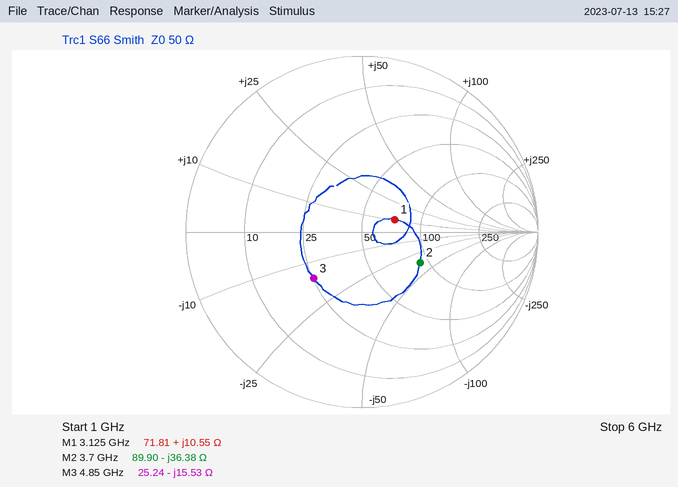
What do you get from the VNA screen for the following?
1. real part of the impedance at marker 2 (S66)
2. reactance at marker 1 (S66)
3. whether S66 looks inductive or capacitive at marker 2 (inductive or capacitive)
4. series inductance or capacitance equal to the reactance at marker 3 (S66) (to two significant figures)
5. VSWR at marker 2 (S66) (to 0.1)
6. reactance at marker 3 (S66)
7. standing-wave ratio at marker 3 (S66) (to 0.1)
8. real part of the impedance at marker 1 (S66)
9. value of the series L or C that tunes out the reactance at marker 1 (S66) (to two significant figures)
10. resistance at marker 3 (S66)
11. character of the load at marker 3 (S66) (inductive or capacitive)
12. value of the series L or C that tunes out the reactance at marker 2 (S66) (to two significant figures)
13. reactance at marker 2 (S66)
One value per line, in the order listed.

89.90 Ω
+10.55 Ω
capacitive
2.1 pF
2.2
-15.53 Ω
2.2
71.81 Ω
4.8 pF
25.24 Ω
capacitive
1.6 nH
-36.38 Ω
